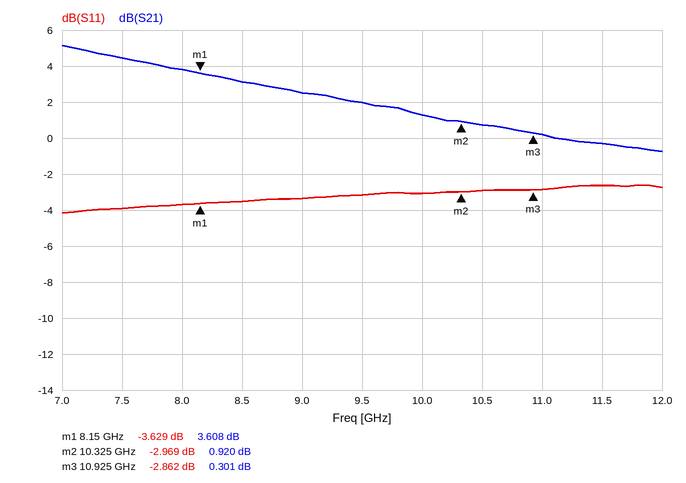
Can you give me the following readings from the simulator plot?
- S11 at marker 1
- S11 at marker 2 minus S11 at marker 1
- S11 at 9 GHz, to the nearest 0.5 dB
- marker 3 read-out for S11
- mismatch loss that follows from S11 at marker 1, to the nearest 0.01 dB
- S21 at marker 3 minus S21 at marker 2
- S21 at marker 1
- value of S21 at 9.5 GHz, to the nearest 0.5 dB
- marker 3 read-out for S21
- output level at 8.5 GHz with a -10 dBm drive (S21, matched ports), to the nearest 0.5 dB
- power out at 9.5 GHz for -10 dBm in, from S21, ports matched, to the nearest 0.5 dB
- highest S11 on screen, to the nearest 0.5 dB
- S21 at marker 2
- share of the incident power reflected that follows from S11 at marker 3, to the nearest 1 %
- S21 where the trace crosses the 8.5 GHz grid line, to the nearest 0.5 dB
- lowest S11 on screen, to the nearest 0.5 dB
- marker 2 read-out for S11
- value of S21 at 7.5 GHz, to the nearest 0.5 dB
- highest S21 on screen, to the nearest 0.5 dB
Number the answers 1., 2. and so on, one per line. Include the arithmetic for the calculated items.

1. -3.629 dB
2. -2.969 − (-3.629) = 0.660 dB
3. -3.5 dB
4. -2.862 dB
5. −10 log10(1 − 10^(-3.629/10)) ≈ 2.47 dB
6. 0.301 − (0.92) = -0.619 dB
7. 3.608 dB
8. 2.0 dB
9. 0.301 dB
10. -10 dBm + (3.0 dB) = -7.0 dBm
11. -10 dBm + (2.0 dB) = -8.0 dBm
12. -2.5 dB
13. 0.920 dB
14. 10^(-2.862/10) ≈ 52 %
15. 3.0 dB
16. -4.0 dB
17. -2.969 dB
18. 4.5 dB
19. 5.0 dB
